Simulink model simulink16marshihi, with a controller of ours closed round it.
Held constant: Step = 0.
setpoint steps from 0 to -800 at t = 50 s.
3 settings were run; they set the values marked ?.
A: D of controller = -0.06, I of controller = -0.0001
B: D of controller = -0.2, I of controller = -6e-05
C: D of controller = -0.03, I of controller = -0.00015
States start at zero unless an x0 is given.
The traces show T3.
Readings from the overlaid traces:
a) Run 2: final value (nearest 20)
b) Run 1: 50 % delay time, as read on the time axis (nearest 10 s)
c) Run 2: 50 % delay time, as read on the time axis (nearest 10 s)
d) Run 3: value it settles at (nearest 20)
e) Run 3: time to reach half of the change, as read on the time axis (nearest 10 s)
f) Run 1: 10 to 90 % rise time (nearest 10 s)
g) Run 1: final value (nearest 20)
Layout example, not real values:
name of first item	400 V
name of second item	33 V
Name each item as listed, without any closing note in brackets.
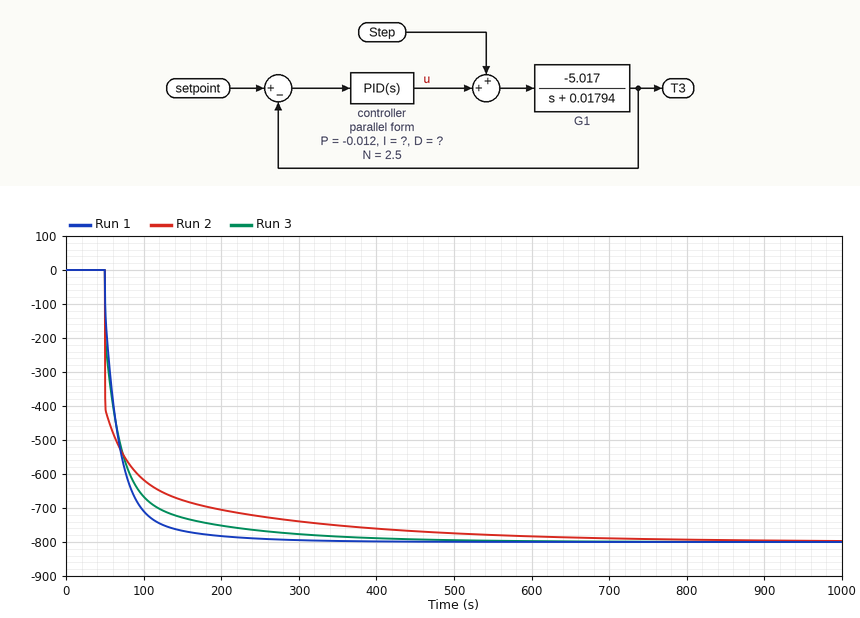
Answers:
Run 2: final value	-800
Run 1: 50 % delay time, as read on the time axis	60 s
Run 2: 50 % delay time, as read on the time axis	50 s
Run 3: value it settles at	-800
Run 3: time to reach half of the change, as read on the time axis	60 s
Run 1: 10 to 90 % rise time	50 s
Run 1: final value	-800
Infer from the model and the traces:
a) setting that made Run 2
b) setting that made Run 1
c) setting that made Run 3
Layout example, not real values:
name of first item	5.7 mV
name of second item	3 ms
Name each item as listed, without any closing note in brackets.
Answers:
setting that made Run 2	B
setting that made Run 1	C
setting that made Run 3	A
